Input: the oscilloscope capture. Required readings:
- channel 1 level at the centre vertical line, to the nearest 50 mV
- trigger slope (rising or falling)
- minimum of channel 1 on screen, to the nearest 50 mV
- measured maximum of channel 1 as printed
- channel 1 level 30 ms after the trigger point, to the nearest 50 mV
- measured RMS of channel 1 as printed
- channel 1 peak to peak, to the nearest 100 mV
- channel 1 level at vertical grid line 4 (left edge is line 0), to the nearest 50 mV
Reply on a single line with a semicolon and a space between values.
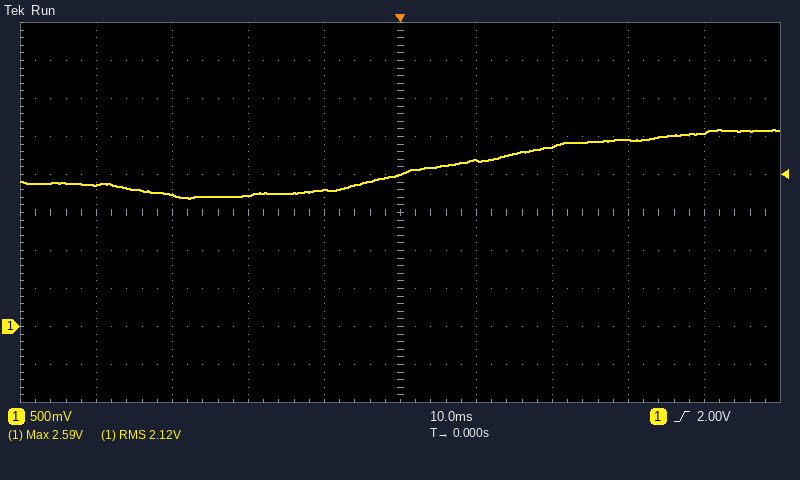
2.00 V; rising; 1.70 V; 2.59 V; 2.45 V; 2.12 V; 900 mV; 1.80 V
